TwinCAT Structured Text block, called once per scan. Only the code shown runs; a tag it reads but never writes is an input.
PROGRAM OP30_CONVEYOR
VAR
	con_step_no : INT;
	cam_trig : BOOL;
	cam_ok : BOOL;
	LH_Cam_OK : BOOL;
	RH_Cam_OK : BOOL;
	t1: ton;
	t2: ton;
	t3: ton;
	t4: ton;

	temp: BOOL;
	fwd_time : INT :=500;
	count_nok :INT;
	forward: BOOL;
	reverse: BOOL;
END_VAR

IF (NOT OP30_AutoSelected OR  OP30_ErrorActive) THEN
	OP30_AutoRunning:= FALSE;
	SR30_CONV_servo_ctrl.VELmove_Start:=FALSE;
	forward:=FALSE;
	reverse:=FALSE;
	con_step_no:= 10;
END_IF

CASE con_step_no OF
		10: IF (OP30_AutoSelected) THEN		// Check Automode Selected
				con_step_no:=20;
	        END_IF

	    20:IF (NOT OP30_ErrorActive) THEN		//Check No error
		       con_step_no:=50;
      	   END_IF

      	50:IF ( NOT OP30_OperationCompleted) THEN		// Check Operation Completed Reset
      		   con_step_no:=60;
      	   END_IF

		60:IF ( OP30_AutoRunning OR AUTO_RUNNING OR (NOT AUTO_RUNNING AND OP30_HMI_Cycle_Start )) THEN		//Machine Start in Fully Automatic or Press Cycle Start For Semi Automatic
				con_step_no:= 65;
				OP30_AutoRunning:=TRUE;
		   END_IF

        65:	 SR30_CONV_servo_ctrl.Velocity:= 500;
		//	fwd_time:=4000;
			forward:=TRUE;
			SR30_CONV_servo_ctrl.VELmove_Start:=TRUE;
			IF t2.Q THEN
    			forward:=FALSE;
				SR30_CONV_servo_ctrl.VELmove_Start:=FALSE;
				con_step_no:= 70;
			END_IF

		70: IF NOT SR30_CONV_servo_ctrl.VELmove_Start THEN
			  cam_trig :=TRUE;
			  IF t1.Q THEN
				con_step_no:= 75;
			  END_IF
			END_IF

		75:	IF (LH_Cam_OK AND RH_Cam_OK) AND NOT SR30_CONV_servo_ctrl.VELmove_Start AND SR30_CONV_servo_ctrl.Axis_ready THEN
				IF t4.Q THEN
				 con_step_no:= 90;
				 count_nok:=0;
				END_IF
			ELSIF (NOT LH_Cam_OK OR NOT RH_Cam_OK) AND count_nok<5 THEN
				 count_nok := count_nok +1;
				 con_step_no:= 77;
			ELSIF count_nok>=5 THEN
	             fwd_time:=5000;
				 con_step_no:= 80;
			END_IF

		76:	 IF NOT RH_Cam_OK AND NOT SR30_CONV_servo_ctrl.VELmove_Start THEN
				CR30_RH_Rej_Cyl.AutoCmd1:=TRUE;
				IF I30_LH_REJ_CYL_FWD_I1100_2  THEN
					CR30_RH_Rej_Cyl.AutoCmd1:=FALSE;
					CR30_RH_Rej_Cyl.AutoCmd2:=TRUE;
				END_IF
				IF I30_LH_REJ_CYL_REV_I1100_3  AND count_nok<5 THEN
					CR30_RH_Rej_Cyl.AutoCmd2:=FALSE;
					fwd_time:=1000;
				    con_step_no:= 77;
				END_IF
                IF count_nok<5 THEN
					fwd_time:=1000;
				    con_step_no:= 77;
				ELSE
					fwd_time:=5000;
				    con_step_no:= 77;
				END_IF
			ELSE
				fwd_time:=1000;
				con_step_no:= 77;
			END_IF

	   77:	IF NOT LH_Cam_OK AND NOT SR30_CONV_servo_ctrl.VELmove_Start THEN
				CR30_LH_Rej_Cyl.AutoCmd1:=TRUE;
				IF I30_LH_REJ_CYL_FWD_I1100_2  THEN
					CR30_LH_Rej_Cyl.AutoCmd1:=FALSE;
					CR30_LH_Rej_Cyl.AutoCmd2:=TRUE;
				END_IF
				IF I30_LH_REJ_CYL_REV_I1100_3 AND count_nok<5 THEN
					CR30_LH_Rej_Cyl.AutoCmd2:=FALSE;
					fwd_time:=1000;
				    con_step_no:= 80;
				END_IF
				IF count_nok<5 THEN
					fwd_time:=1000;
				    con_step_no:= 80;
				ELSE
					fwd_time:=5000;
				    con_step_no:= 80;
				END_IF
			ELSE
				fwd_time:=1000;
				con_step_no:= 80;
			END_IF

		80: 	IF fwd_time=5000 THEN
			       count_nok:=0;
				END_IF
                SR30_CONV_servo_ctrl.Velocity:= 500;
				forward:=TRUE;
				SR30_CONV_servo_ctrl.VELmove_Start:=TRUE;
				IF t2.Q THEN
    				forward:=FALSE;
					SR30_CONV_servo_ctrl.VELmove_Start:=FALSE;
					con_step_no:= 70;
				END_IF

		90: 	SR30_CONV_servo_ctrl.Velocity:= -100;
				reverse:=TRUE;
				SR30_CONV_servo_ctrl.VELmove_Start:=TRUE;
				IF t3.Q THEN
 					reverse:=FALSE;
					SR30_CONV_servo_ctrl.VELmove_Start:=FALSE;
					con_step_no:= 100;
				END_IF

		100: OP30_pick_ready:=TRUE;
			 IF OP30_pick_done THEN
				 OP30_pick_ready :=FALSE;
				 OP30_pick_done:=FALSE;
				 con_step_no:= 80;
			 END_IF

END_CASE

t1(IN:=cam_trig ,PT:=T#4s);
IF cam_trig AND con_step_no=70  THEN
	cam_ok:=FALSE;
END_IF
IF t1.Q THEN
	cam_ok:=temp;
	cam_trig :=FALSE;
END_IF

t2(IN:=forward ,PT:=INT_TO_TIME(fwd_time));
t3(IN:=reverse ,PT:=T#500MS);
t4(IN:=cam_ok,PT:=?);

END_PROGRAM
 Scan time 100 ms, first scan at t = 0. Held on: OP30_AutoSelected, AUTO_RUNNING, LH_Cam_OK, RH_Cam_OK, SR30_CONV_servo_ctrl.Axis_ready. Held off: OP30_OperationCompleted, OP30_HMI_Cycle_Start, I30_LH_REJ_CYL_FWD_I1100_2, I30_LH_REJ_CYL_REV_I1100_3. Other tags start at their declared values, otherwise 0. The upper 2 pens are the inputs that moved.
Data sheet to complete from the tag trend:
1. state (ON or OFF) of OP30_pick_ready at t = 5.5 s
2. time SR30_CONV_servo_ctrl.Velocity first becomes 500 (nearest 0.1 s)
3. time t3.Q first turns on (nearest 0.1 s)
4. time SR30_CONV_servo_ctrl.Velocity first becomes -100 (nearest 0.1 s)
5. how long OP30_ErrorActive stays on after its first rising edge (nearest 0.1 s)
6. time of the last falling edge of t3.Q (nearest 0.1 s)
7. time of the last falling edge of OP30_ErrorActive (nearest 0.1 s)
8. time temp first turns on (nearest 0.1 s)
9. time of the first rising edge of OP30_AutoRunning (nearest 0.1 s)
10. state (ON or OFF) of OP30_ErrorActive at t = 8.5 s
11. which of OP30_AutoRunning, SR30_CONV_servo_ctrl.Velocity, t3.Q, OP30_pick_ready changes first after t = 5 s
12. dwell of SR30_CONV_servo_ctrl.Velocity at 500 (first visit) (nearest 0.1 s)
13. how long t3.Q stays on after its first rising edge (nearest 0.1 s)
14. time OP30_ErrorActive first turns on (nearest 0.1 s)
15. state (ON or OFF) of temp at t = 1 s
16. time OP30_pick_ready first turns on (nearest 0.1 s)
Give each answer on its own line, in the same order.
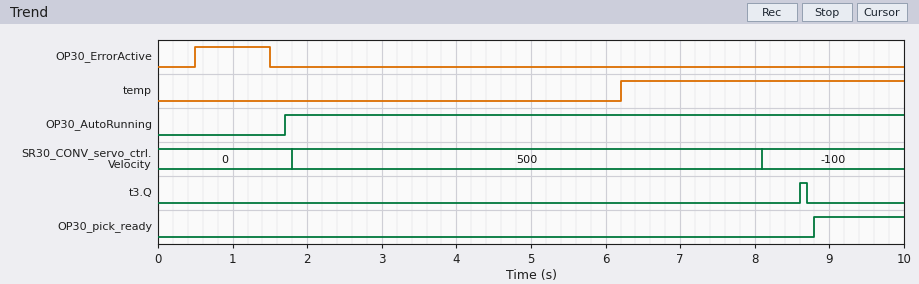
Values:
OFF
1.8 s
8.6 s
8.1 s
1.0 s
8.7 s
1.5 s
6.2 s
1.7 s
OFF
SR30_CONV_servo_ctrl.Velocity
6.3 s
0.1 s
0.5 s
OFF
8.8 s
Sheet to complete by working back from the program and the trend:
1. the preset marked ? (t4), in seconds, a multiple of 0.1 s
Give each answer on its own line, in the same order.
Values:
1.4 s
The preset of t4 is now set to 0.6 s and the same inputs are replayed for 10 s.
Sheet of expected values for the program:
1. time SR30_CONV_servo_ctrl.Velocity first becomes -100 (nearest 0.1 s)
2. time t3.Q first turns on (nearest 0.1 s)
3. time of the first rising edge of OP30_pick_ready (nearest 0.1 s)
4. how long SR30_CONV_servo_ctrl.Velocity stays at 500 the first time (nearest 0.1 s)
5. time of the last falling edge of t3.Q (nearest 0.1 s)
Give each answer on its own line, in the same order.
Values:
7.3 s
7.8 s
8.0 s
5.5 s
7.9 s
